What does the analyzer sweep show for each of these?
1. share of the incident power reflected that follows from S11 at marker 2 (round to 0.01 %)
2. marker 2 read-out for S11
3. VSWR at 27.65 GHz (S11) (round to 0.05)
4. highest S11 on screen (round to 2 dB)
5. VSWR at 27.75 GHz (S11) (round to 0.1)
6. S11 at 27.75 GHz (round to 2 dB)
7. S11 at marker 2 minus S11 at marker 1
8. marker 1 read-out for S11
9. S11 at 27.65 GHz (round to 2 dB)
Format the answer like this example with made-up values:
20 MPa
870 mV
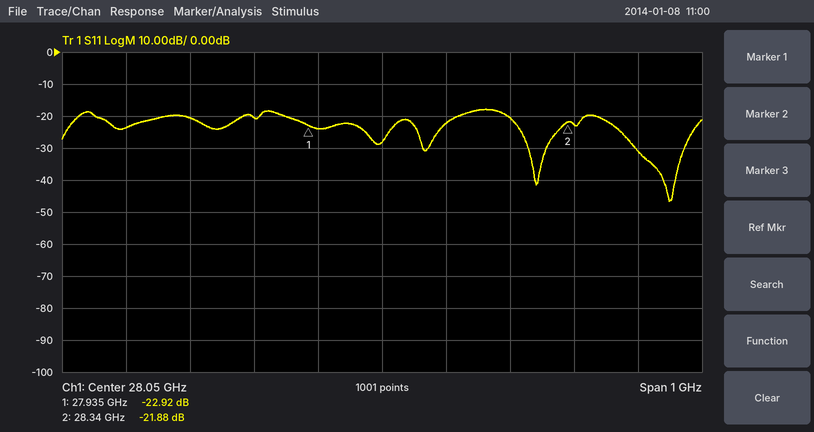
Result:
0.65 %
-21.88 dB
1.15
-18 dB
1.2
-20 dB
1.04 dB
-22.92 dB
-24 dB
